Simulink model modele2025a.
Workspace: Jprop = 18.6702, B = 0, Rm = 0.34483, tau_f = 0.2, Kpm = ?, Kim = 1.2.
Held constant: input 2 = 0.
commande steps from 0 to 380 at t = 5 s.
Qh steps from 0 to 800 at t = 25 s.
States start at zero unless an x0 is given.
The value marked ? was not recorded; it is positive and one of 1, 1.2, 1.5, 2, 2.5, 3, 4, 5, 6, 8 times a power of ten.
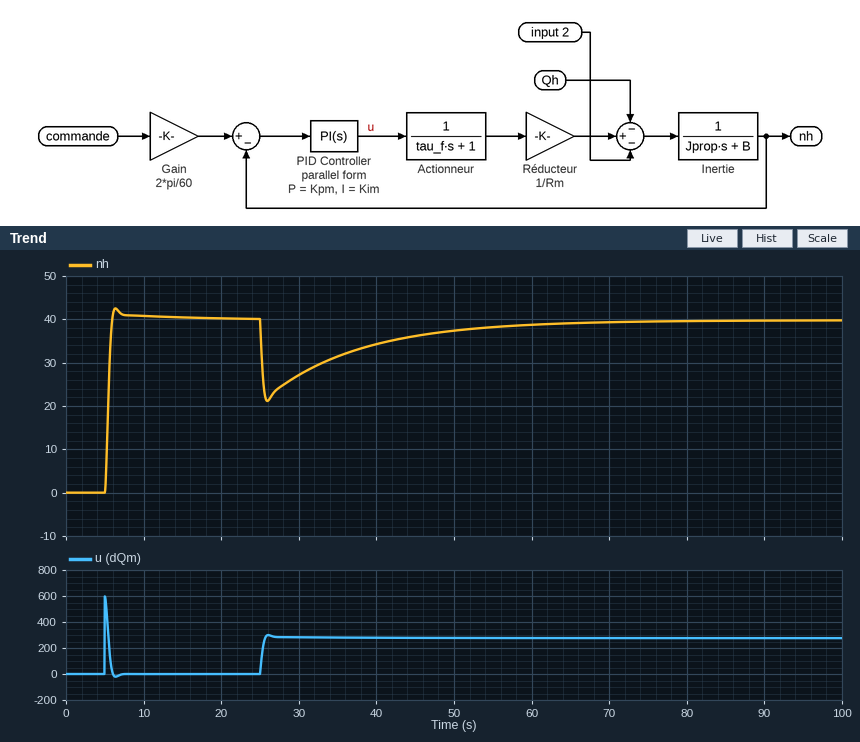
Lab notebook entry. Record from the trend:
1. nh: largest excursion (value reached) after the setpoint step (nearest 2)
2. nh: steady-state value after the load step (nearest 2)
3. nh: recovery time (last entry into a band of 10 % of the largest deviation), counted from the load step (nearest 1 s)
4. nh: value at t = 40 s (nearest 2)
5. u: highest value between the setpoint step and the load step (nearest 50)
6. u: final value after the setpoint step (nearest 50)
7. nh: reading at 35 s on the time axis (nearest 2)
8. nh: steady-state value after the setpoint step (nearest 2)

42
40
28 s
34
600
0
32
40
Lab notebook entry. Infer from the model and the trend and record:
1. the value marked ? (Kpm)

15
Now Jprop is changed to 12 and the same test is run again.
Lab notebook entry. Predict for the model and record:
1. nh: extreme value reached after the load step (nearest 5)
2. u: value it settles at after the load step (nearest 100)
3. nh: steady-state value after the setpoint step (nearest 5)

20
300
40
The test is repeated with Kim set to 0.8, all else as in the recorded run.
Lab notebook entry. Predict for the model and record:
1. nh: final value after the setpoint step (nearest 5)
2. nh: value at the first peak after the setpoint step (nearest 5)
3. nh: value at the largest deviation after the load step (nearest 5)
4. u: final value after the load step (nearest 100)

40
40
20
300
